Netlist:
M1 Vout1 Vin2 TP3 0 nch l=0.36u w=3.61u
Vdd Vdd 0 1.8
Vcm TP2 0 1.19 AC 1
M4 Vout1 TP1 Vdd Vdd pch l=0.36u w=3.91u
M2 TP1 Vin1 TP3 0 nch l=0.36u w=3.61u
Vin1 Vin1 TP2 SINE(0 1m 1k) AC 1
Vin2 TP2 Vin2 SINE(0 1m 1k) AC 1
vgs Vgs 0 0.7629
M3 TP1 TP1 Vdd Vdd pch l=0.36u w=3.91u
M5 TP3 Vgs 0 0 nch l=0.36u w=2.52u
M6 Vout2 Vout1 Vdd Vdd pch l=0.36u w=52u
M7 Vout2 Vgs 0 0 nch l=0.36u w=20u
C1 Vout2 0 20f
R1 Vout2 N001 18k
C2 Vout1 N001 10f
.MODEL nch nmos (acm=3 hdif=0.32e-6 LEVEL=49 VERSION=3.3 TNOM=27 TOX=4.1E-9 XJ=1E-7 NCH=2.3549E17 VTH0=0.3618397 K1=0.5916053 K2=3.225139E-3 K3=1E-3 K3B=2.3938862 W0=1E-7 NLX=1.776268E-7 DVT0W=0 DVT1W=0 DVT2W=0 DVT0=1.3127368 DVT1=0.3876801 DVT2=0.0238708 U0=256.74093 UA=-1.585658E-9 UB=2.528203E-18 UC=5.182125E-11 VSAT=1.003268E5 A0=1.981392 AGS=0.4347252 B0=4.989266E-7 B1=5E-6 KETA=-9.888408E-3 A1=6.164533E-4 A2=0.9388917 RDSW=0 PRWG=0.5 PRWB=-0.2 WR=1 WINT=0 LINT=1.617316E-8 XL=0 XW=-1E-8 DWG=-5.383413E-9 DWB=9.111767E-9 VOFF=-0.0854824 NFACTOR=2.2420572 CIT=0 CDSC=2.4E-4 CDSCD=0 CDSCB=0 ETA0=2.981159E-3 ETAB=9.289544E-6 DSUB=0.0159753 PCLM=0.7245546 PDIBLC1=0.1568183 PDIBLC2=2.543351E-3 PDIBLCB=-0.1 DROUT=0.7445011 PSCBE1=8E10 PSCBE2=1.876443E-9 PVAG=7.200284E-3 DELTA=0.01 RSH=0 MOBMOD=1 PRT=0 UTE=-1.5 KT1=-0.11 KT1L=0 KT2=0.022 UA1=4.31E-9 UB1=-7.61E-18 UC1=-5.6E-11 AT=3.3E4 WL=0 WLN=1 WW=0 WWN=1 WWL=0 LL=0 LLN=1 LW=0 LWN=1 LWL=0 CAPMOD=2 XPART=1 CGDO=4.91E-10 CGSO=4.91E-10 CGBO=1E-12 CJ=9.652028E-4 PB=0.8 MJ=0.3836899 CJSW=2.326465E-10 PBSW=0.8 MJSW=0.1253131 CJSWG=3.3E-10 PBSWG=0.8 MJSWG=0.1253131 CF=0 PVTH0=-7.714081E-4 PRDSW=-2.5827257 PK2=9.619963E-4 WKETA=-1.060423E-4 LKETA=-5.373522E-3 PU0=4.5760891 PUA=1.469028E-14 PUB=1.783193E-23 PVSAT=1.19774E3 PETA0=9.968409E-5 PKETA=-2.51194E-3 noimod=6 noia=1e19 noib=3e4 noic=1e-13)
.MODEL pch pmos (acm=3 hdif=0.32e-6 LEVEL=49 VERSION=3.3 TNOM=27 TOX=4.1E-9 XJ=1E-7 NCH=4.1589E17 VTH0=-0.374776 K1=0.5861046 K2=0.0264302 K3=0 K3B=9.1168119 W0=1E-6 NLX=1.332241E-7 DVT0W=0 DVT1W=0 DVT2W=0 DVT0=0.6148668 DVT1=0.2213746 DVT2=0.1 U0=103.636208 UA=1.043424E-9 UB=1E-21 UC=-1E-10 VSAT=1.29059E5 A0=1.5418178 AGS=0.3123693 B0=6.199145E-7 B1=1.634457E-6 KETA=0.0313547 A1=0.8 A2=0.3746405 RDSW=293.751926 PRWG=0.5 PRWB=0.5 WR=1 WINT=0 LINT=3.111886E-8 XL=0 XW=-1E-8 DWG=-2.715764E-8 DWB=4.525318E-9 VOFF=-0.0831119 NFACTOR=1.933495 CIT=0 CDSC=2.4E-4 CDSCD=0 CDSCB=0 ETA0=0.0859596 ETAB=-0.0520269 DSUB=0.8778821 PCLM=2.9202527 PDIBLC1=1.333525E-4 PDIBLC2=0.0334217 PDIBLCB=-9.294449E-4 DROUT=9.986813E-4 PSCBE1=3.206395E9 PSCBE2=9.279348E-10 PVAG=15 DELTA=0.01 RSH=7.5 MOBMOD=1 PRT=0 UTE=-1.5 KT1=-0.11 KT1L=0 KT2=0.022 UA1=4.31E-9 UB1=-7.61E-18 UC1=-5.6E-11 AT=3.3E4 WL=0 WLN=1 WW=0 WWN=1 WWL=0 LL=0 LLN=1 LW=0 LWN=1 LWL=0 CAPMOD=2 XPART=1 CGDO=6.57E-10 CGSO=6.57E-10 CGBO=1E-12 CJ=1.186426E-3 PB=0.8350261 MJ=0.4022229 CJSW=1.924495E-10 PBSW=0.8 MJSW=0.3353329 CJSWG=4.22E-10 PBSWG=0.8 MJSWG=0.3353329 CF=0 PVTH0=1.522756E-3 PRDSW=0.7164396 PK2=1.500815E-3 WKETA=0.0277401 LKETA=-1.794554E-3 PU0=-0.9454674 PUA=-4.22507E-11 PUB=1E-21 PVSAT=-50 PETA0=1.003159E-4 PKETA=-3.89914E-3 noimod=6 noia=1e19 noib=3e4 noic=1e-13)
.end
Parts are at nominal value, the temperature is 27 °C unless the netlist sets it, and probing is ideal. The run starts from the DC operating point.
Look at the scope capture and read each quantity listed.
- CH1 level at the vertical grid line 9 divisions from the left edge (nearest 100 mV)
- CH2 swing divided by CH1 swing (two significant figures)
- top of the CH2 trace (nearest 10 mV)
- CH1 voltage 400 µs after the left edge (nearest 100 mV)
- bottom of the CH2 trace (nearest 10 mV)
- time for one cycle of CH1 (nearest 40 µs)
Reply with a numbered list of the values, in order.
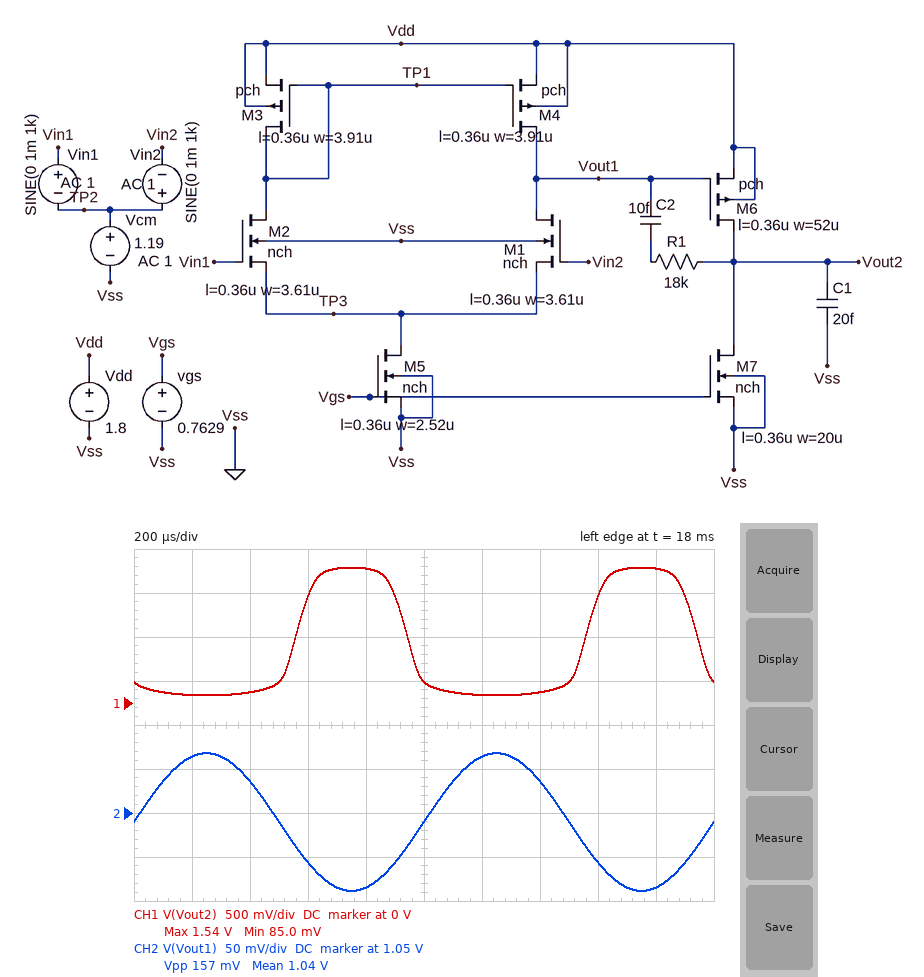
1. 1.5 V
2. 0.11
3. 1.12 V
4. 100 mV
5. 960 mV
6. 1.00 ms
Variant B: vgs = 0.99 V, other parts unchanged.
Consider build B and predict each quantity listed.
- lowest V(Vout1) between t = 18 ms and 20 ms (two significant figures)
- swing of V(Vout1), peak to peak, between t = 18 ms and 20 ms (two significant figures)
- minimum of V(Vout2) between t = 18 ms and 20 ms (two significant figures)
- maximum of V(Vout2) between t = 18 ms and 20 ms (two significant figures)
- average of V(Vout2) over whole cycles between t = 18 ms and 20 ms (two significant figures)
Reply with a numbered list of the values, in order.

1. 770 mV
2. 110 mV
3. 180 mV
4. 440 mV
5. 280 mV
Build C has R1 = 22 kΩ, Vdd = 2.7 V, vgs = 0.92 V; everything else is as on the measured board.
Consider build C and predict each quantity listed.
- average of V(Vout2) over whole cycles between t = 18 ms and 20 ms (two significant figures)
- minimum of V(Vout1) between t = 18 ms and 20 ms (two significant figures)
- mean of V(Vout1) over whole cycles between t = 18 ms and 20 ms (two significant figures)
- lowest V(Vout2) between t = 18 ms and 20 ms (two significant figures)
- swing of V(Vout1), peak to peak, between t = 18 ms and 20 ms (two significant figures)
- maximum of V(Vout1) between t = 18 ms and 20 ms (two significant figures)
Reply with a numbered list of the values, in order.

1. 690 mV
2. 1.7 V
3. 1.8 V
4. 160 mV
5. 160 mV
6. 1.9 V
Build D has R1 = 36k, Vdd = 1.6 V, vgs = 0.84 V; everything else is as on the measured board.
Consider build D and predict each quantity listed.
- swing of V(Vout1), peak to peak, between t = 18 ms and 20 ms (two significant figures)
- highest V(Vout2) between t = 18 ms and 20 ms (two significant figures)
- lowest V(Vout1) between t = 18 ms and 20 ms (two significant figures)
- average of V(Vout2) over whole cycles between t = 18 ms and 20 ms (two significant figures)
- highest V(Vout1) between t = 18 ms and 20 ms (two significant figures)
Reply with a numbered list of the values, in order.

1. 110 mV
2. 860 mV
3. 710 mV
4. 360 mV
5. 820 mV
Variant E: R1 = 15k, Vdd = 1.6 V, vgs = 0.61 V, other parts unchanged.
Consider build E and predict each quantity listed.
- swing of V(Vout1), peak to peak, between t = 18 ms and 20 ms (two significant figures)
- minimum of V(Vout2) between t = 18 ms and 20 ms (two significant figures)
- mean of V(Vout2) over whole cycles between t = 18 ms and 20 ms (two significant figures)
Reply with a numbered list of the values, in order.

1. 170 mV
2. 24 mV
3. 700 mV
